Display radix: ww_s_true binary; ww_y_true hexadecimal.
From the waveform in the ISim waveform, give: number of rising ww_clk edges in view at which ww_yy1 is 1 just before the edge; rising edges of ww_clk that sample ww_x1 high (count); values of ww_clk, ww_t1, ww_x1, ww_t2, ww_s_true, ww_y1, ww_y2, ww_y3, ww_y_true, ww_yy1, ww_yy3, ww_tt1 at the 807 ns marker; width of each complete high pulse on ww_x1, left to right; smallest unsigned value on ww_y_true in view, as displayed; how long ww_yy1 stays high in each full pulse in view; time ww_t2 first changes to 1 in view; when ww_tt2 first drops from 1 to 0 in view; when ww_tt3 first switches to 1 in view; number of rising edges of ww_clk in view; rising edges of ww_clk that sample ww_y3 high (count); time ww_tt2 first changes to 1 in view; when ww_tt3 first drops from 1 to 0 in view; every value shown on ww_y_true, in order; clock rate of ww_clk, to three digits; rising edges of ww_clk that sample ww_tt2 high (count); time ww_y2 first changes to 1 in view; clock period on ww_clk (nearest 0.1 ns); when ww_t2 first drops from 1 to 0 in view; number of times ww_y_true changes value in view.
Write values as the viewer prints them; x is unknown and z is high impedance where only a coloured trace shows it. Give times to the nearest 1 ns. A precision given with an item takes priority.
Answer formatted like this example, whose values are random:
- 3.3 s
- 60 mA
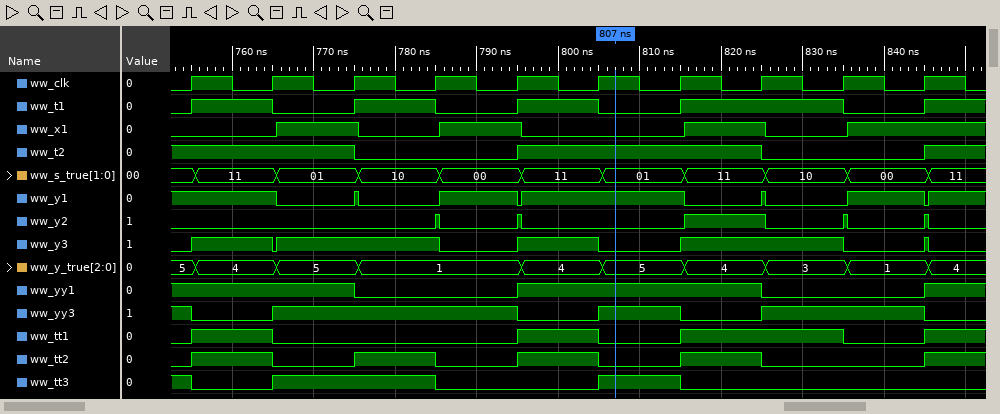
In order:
- 6
- 4
- ww_clk=1, ww_t1=0, ww_x1=0, ww_t2=1, ww_s_true=01, ww_y1=1, ww_y2=0, ww_y3=0, ww_y_true=5, ww_yy1=1, ww_yy3=1, ww_tt1=0
- 10 ns, 10 ns, 10 ns
- 1
- 30 ns
- 795 ns
- 765 ns
- 765 ns
- 10
- 6
- 755 ns
- 755 ns
- 5, 4, 5, 1, 4, 5, 4, 3, 1, 4
- 100 MHz
- 4
- 785 ns
- 10 ns
- 775 ns
- 9
